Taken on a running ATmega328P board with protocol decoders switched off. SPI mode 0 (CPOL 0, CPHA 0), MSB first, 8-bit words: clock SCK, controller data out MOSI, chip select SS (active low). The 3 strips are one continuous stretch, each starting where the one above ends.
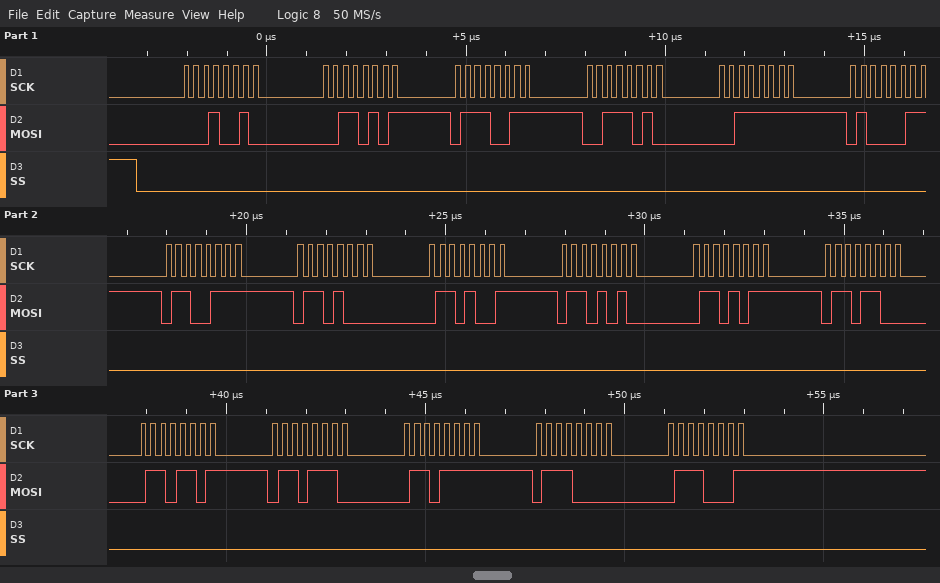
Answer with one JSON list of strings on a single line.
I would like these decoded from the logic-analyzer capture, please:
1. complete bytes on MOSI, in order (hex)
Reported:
["12 35 73 3A 3F 43 67 68 69 6A 6B 6C 6D 6E 6F 70 71"]
